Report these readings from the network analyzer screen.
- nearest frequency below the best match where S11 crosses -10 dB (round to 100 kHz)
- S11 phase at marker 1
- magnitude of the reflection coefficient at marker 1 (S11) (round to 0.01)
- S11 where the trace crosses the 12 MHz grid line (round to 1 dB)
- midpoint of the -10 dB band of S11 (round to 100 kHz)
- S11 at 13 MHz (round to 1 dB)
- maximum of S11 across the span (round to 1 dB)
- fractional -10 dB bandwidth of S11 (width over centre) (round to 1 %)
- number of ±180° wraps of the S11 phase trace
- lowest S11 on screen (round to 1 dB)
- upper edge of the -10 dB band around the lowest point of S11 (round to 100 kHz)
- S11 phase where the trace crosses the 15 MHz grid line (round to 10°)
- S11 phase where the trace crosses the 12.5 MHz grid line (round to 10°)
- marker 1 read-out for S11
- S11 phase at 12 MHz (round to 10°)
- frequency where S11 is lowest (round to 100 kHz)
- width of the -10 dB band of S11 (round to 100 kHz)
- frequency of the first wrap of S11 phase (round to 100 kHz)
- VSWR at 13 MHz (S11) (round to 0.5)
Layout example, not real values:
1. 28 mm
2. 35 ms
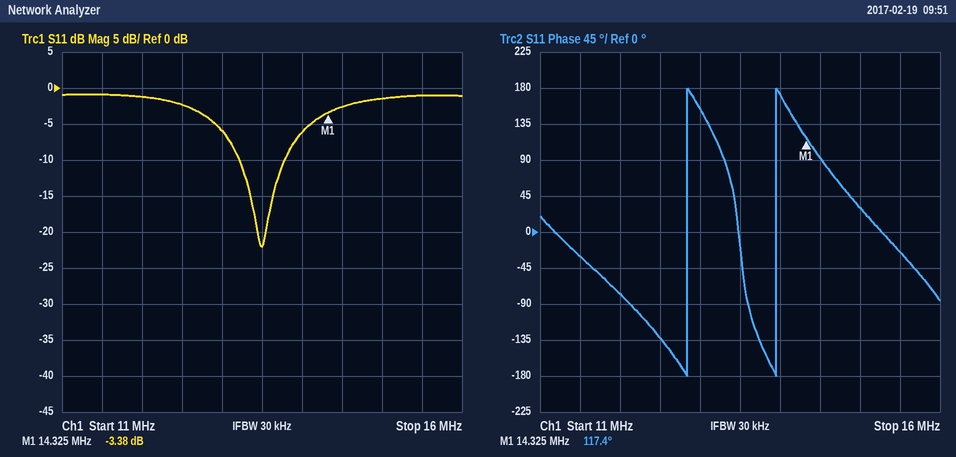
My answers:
1. 13.2 MHz
2. 117.4°
3. 0.68
4. -1 dB
5. 13.5 MHz
6. -6 dB
7. -1 dB
8. 4 %
9. 2
10. -22 dB
11. 13.8 MHz
12. 30°
13. -130°
14. -3.38 dB
15. -80°
16. 13.5 MHz
17. 600 kHz
18. 12.8 MHz
19. 3.0
